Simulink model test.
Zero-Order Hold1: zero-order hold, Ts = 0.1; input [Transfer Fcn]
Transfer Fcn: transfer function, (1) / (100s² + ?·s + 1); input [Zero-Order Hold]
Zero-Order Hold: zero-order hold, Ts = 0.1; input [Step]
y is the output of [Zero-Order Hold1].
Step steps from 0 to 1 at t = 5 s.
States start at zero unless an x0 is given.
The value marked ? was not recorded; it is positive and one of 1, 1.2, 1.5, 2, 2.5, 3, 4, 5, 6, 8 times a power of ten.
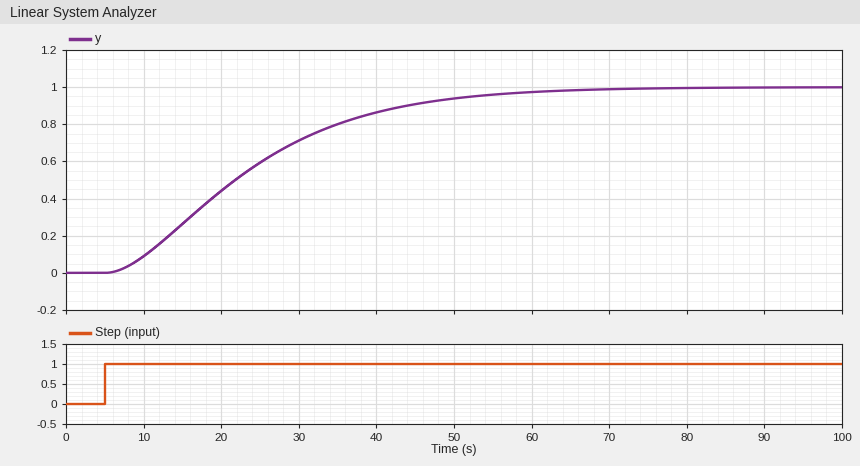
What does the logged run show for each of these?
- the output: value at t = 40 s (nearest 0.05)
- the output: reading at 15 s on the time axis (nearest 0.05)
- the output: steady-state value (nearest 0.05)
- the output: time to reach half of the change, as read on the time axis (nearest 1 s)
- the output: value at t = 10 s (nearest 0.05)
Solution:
0.85
0.25
1.00
22 s
0.10
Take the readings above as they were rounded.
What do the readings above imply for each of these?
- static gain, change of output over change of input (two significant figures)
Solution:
1.0
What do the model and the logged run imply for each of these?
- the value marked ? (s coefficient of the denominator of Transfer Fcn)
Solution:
20
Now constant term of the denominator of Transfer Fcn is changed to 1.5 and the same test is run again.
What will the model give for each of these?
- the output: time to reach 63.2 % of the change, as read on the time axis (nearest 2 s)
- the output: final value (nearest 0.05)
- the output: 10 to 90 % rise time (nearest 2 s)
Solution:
20 s
0.65
20 s
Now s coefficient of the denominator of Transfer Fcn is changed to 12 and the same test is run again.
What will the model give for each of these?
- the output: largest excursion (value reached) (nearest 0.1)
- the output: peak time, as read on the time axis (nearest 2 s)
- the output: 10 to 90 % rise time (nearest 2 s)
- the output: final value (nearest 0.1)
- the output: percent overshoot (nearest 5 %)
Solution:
1.1
44 s
18 s
1.0
10 %
